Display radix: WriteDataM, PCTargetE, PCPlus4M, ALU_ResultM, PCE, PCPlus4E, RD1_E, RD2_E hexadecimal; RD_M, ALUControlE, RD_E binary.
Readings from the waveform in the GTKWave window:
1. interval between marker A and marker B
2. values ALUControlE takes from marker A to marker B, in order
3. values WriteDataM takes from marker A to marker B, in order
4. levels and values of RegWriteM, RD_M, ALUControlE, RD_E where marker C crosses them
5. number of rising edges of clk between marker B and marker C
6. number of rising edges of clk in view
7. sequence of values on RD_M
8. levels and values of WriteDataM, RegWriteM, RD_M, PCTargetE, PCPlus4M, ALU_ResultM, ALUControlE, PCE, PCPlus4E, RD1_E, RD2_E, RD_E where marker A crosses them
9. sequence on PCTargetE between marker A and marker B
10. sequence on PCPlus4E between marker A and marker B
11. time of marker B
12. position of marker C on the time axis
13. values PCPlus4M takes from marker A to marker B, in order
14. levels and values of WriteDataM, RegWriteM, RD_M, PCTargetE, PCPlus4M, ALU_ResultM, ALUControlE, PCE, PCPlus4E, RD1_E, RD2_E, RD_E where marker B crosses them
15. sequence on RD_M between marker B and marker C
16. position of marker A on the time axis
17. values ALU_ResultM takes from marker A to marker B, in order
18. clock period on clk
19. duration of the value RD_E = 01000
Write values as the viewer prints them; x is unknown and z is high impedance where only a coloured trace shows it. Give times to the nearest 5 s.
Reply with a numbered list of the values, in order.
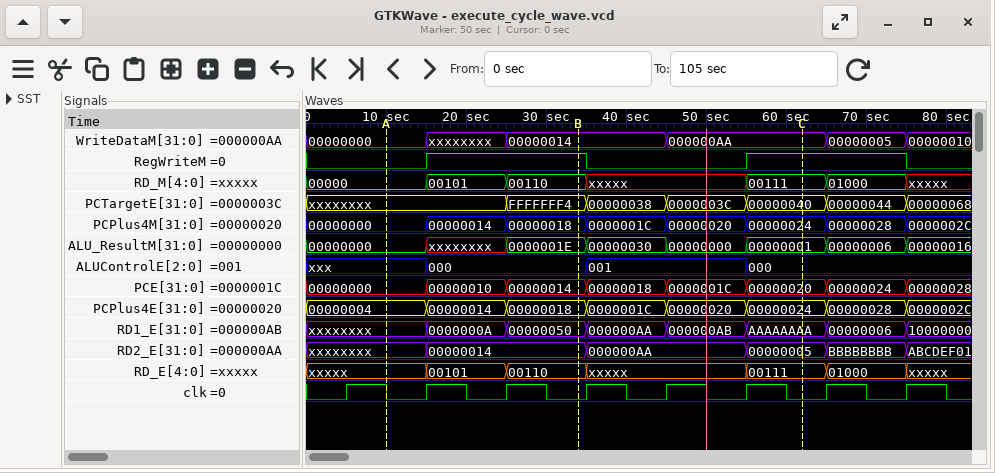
1. 25 s
2. xxx, 000
3. 00000000, xxxxxxxx, 00000014
4. RegWriteM=1, RD_M=00111, ALUControlE=000, RD_E=00111
5. 3
6. 8
7. 00000, 00101, 00110, xxxxx, 00111, 01000, xxxxx
8. WriteDataM=00000000, RegWriteM=0, RD_M=00000, PCTargetE=xxxxxxxx, PCPlus4M=00000000, ALU_ResultM=00000000, ALUControlE=xxx, PCE=00000000, PCPlus4E=00000004, RD1_E=xxxxxxxx, RD2_E=xxxxxxxx, RD_E=xxxxx
9. xxxxxxxx, FFFFFFF4
10. 00000004, 00000014, 00000018
11. 35 s
12. 60 s
13. 00000000, 00000014, 00000018
14. WriteDataM=00000014, RegWriteM=1, RD_M=00110, PCTargetE=FFFFFFF4, PCPlus4M=00000018, ALU_ResultM=0000001E, ALUControlE=000, PCE=00000014, PCPlus4E=00000018, RD1_E=00000050, RD2_E=00000014, RD_E=00110
15. 00110, xxxxx, 00111
16. 10 s
17. 00000000, xxxxxxxx, 0000001E
18. 10 s
19. 10 s
